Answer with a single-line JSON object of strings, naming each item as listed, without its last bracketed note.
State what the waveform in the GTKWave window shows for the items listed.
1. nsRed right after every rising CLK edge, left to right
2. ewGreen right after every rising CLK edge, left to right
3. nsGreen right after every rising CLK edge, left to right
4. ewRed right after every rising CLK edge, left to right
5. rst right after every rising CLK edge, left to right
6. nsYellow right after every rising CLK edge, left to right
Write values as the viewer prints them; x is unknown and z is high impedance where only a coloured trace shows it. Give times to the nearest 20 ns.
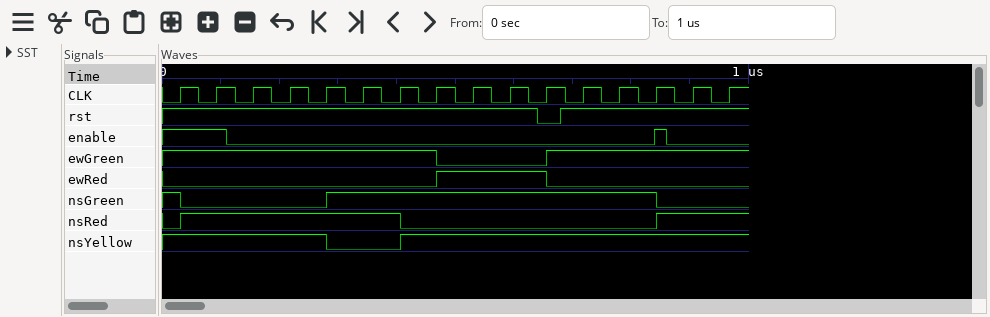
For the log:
{"nsRed right after every rising CLK edge, left to right": "1 1 1 1 1 1 0 0 0 0 0 0 0 1 1 1", "ewGreen right after every rising CLK edge, left to right": "1 1 1 1 1 1 1 0 0 0 1 1 1 1 1 1", "nsGreen right after every rising CLK edge, left to right": "0 0 0 0 1 1 1 1 1 1 1 1 1 0 0 0", "ewRed right after every rising CLK edge, left to right": "0 0 0 0 0 0 0 1 1 1 0 0 0 0 0 0", "rst right after every rising CLK edge, left to right": "1 1 1 1 1 1 1 1 1 1 0 1 1 1 1 1", "nsYellow right after every rising CLK edge, left to right": "1 1 1 1 0 0 1 1 1 1 1 1 1 1 1 1"}
